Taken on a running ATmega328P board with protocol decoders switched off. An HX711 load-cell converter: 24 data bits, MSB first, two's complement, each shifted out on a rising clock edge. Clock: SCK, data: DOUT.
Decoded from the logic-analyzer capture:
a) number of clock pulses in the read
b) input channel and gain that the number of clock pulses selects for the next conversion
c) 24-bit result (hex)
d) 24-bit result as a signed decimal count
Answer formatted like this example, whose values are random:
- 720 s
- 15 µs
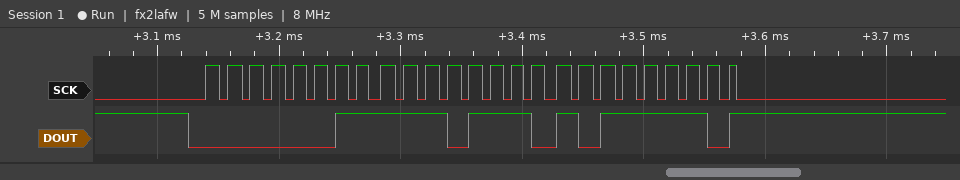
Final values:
- 25
- channel A, gain 128
- 0x03EEBE
- 257726
